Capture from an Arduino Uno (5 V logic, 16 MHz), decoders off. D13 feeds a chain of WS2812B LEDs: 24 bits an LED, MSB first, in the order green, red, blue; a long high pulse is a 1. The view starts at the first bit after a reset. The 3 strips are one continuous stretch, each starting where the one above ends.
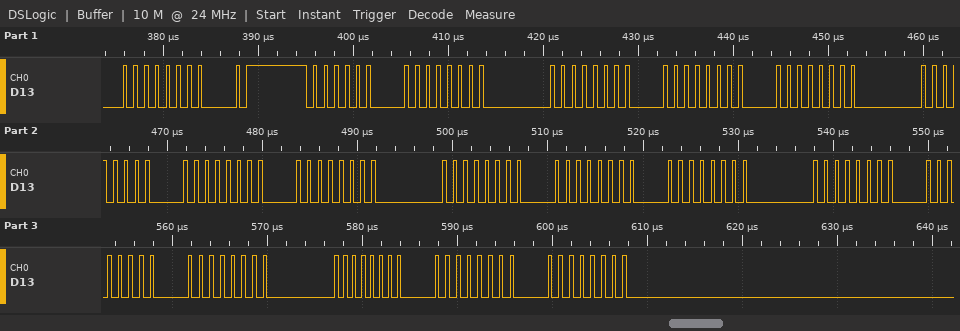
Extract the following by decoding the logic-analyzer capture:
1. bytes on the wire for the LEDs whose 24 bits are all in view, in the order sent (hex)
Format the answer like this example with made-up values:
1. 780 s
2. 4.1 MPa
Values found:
1. 00 40 00 00 00 00 00 00 00 00 00 00 00 00 00 00 00 00
